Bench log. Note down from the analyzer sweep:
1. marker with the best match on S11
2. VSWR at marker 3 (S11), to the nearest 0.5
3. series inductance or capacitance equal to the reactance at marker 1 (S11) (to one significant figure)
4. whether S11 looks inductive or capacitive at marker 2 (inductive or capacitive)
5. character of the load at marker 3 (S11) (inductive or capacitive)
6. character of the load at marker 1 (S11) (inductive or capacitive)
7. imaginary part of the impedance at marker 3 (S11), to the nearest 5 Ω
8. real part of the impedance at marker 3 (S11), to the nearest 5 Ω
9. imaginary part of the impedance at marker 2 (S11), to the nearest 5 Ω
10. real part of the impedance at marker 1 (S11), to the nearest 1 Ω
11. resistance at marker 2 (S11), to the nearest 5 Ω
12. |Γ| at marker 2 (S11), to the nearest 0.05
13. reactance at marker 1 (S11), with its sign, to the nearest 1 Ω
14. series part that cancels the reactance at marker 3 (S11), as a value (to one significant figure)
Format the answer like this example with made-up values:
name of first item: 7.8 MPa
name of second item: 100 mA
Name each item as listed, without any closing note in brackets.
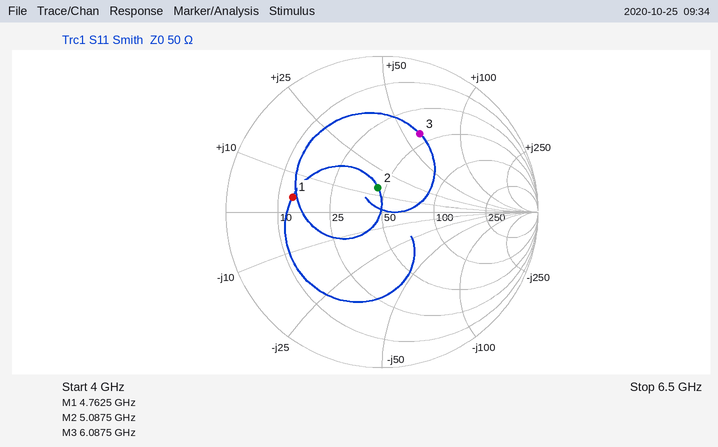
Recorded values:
marker with the best match on S11: marker 2
VSWR at marker 3 (S11), to the nearest 0.5: 3.5
series inductance or capacitance equal to the reactance at marker 1 (S11): 100 pH
whether S11 looks inductive or capacitive at marker 2: inductive
character of the load at marker 3 (S11): inductive
character of the load at marker 1 (S11): inductive
imaginary part of the impedance at marker 3 (S11), to the nearest 5 Ω: +60 Ω
real part of the impedance at marker 3 (S11), to the nearest 5 Ω: 40 Ω
imaginary part of the impedance at marker 2 (S11), to the nearest 5 Ω: +15 Ω
real part of the impedance at marker 1 (S11), to the nearest 1 Ω: 13 Ω
resistance at marker 2 (S11), to the nearest 5 Ω: 45 Ω
|Γ| at marker 2 (S11), to the nearest 0.05: 0.15
reactance at marker 1 (S11), with its sign, to the nearest 1 Ω: +4 Ω
series part that cancels the reactance at marker 3 (S11), as a value: 400 fF
